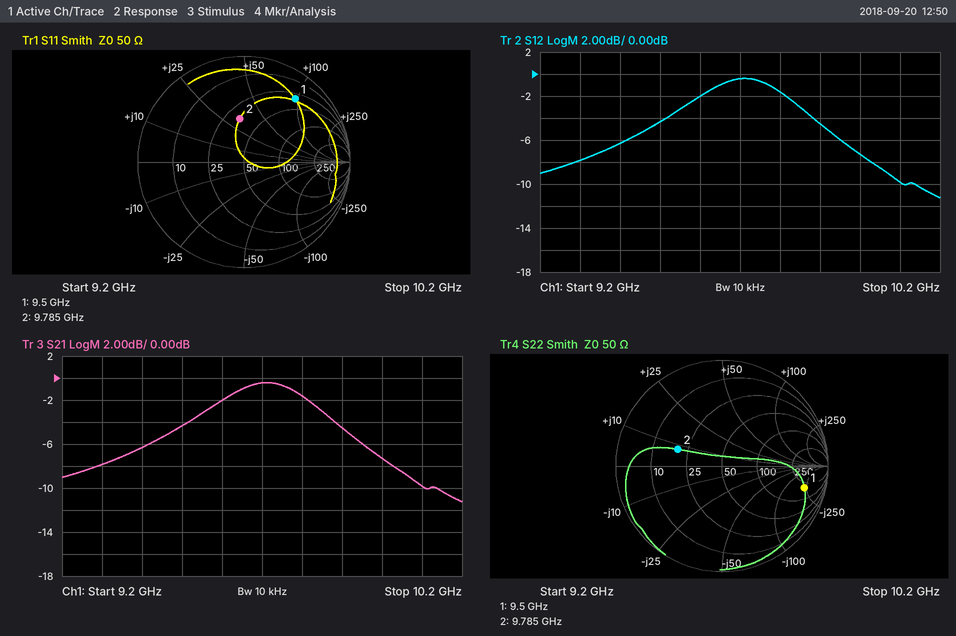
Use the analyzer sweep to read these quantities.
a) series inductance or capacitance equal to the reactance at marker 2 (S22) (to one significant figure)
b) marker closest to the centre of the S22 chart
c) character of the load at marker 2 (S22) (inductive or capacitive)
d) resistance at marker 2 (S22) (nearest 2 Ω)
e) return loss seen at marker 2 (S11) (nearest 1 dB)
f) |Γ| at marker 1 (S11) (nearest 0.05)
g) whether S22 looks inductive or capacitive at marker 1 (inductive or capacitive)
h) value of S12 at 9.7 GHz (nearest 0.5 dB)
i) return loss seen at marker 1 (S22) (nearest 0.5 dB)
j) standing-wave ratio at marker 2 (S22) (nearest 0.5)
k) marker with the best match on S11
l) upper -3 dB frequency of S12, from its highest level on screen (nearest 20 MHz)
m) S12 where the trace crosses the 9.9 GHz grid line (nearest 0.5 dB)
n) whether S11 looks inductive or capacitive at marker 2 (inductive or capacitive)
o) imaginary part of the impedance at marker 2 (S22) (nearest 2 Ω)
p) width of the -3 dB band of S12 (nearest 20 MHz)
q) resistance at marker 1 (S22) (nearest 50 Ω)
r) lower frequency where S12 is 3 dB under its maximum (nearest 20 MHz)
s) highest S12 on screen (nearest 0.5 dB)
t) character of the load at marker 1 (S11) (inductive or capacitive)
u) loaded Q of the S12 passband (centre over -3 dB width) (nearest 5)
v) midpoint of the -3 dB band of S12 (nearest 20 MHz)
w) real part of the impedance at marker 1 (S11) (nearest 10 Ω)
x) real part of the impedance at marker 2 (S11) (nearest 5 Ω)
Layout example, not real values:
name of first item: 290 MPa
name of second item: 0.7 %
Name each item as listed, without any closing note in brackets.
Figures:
series inductance or capacitance equal to the reactance at marker 2 (S22): 100 pH
marker closest to the centre of the S22 chart: marker 2
character of the load at marker 2 (S22): inductive
resistance at marker 2 (S22): 20 Ω
return loss seen at marker 2 (S11): 8 dB
|Γ| at marker 1 (S11): 0.75
whether S22 looks inductive or capacitive at marker 1: capacitive
value of S12 at 9.7 GHz: -0.5 dB
return loss seen at marker 1 (S22): 2.0 dB
standing-wave ratio at marker 2 (S22): 2.5
marker with the best match on S11: marker 2
upper -3 dB frequency of S12, from its highest level on screen: 9.86 GHz
S12 where the trace crosses the 9.9 GHz grid line: -4.5 dB
whether S11 looks inductive or capacitive at marker 2: inductive
imaginary part of the impedance at marker 2 (S22): +8 Ω
width of the -3 dB band of S12: 320 MHz
resistance at marker 1 (S22): 200 Ω
lower frequency where S12 is 3 dB under its maximum: 9.54 GHz
highest S12 on screen: -0.5 dB
character of the load at marker 1 (S11): inductive
loaded Q of the S12 passband (centre over -3 dB width): 30
midpoint of the -3 dB band of S12: 9.70 GHz
real part of the impedance at marker 1 (S11): 30 Ω
real part of the impedance at marker 2 (S11): 35 Ω
